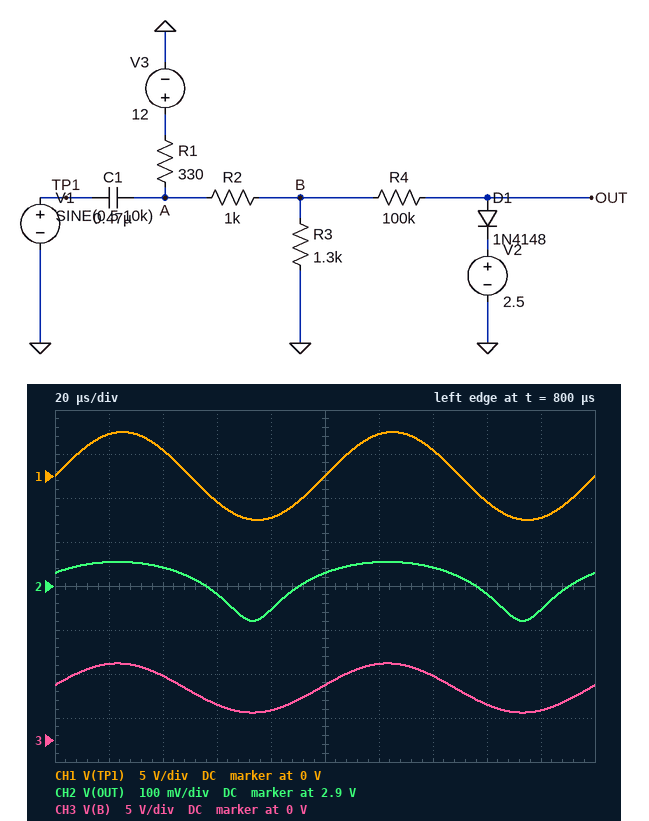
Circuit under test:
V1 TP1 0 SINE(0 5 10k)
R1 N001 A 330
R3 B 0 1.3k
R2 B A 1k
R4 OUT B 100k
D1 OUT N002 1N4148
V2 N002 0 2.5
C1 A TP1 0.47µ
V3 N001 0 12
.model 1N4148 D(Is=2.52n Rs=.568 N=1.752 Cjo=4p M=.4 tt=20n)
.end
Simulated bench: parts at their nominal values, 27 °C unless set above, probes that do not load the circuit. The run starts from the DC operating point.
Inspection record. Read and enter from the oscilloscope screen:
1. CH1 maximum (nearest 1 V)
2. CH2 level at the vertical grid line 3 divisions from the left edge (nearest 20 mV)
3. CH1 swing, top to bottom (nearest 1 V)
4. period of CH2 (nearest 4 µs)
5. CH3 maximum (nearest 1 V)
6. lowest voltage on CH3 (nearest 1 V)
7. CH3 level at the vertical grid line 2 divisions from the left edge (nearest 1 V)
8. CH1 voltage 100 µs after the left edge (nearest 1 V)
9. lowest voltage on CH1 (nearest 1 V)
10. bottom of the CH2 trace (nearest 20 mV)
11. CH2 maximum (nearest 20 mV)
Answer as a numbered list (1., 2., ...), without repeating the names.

1. 5 V
2. 2.88 V
3. 10 V
4. 100 µs
5. 9 V
6. 3 V
7. 7 V
8. 0 V
9. -5 V
10. 2.82 V
11. 2.96 V
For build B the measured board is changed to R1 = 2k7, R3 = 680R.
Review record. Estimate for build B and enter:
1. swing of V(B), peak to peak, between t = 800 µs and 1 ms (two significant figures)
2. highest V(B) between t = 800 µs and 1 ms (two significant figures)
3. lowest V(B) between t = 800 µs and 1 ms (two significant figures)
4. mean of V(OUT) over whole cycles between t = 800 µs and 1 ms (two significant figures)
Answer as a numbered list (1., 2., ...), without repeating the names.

1. 4.0 V
2. 3.9 V
3. -170 mV
4. 1.6 V
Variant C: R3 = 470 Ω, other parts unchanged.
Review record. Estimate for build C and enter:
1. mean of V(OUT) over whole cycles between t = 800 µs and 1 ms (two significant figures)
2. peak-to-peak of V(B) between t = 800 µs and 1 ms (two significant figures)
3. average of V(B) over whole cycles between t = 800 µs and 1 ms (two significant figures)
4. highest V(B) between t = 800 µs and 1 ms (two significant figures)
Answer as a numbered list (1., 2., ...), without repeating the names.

1. 2.5 V
2. 3.2 V
3. 3.1 V
4. 4.7 V
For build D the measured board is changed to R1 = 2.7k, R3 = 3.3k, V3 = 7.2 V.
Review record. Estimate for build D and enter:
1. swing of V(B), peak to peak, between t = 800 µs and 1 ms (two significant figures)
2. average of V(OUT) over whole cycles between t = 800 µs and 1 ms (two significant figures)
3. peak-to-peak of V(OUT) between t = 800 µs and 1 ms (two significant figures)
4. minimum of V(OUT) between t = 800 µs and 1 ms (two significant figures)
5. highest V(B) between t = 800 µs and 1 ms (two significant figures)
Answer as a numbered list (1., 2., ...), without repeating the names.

1. 7.6 V
2. 1.9 V
3. 3.4 V
4. -480 mV
5. 7.2 V
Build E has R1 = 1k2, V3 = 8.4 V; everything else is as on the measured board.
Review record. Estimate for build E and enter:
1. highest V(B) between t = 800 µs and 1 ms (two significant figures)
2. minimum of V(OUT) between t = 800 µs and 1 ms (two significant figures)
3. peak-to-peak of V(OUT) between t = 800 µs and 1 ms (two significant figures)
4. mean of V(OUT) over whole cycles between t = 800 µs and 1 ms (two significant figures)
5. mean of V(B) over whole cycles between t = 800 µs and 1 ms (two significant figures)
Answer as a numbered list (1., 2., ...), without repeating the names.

1. 5.9 V
2. 280 mV
3. 2.6 V
4. 2.1 V
5. 3.1 V
